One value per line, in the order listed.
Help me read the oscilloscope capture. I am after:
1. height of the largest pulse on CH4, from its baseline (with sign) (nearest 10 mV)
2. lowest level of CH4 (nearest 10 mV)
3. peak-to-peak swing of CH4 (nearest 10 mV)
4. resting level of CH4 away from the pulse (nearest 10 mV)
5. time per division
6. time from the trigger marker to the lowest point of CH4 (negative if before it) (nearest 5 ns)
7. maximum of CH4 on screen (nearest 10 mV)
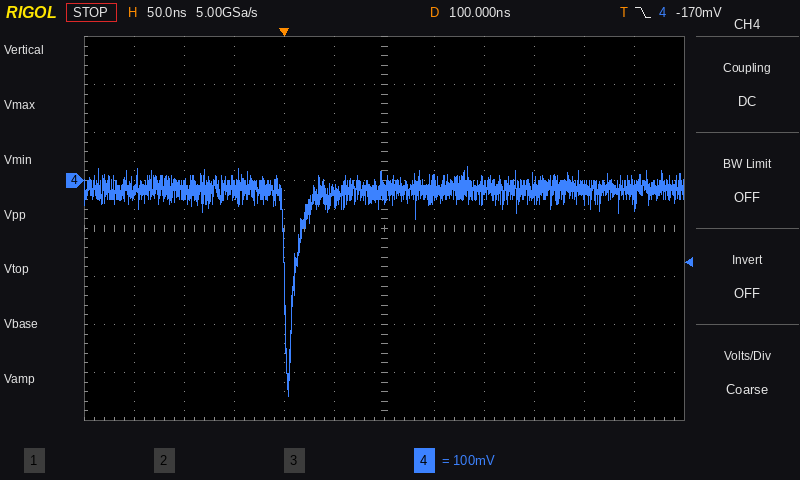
-430 mV
-450 mV
480 mV
-20 mV
50 ns
+5 ns
30 mV
